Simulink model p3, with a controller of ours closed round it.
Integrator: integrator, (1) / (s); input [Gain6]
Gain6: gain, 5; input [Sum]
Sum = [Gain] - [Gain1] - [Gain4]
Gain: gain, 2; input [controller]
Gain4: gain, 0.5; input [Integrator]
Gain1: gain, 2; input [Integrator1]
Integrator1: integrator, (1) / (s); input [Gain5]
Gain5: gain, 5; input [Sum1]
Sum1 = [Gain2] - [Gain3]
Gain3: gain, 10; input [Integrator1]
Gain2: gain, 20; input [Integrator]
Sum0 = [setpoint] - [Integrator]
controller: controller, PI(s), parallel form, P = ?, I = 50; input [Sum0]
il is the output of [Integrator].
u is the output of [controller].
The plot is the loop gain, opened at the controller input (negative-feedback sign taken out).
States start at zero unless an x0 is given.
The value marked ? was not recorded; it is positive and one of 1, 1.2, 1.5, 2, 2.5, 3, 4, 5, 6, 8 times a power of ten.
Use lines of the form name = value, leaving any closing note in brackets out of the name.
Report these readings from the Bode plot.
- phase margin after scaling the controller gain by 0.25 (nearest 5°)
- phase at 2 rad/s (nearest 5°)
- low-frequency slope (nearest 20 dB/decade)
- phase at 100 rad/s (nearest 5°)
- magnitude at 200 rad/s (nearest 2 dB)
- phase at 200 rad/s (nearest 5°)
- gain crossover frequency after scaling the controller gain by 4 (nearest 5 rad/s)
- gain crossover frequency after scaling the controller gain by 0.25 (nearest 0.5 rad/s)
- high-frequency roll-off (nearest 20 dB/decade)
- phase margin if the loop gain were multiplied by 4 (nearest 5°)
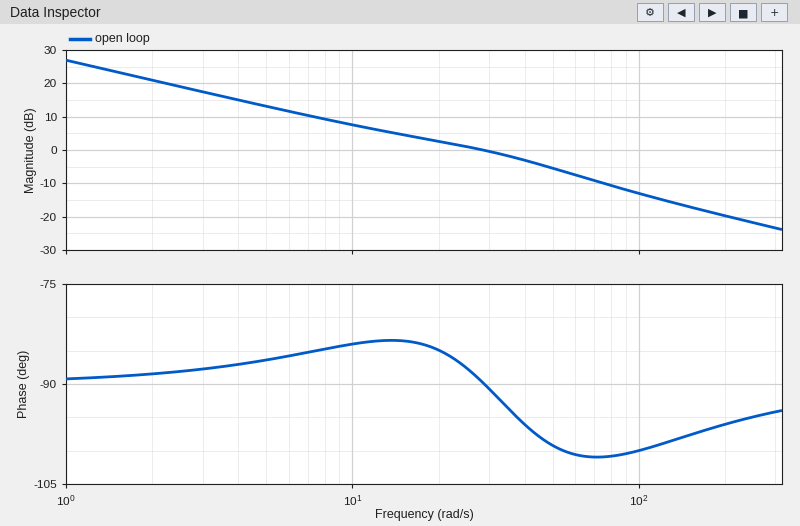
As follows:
phase margin after scaling the controller gain by 0.25 = 95°
phase at 2 rad/s = -90°
low-frequency slope = -20 dB/decade
phase at 100 rad/s = -100°
magnitude at 200 rad/s = -20 dB
phase at 200 rad/s = -95°
gain crossover frequency after scaling the controller gain by 4 = 90 rad/s
gain crossover frequency after scaling the controller gain by 0.25 = 5.5 rad/s
high-frequency roll-off = -20 dB/decade
phase margin if the loop gain were multiplied by 4 = 80°
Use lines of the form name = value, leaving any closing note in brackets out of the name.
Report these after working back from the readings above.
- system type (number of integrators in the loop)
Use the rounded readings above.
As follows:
system type = 1
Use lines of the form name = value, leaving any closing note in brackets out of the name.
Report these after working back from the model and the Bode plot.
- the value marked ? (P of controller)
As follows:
the value marked ? = 2
